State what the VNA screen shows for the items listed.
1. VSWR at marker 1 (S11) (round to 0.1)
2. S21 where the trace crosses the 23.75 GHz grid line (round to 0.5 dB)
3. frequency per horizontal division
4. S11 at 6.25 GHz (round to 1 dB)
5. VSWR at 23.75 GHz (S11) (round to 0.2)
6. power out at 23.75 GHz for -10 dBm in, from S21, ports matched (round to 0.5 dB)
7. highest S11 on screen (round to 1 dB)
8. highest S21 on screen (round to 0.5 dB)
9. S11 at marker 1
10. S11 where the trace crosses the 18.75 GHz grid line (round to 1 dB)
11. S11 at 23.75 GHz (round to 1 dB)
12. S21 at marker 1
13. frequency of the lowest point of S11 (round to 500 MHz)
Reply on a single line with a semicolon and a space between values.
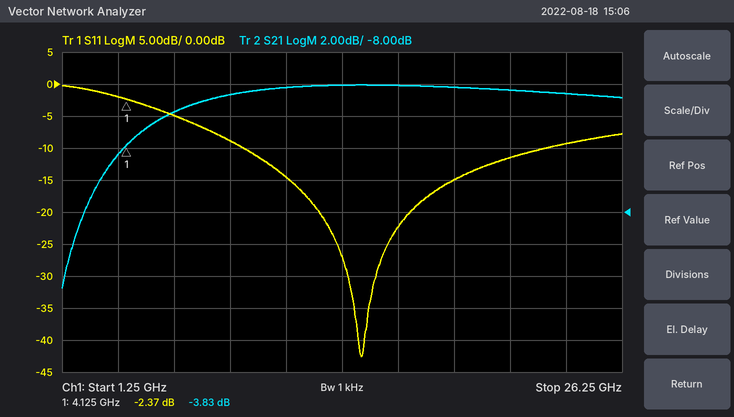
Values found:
7.4; -0.5 dB; 2.5 GHz; -5 dB; 2.0; -10.5 dBm; 0 dB; 0.0 dB; -2.37 dB; -15 dB; -9 dB; -3.83 dB; 14.5 GHz
